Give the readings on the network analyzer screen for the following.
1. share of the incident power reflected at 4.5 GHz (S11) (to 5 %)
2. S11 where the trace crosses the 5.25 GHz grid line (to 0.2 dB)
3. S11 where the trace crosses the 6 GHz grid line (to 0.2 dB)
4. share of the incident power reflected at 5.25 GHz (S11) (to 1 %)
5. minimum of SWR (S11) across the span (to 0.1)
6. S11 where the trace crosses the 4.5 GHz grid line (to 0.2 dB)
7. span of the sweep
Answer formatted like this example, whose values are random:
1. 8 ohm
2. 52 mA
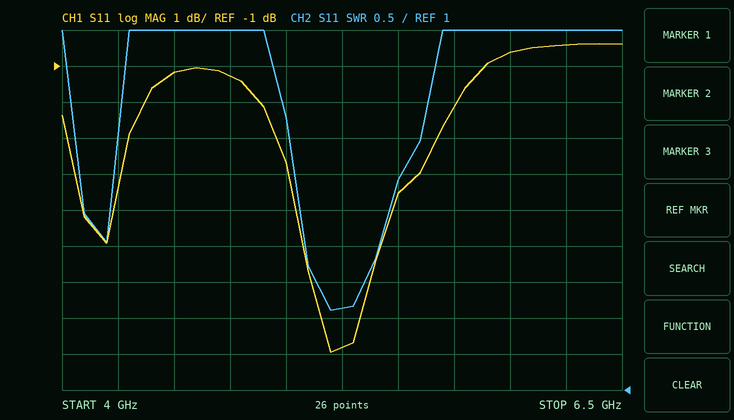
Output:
1. 75 %
2. -8.8 dB
3. -0.6 dB
4. 13 %
5. 2.1
6. -1.2 dB
7. 2.5 GHz
